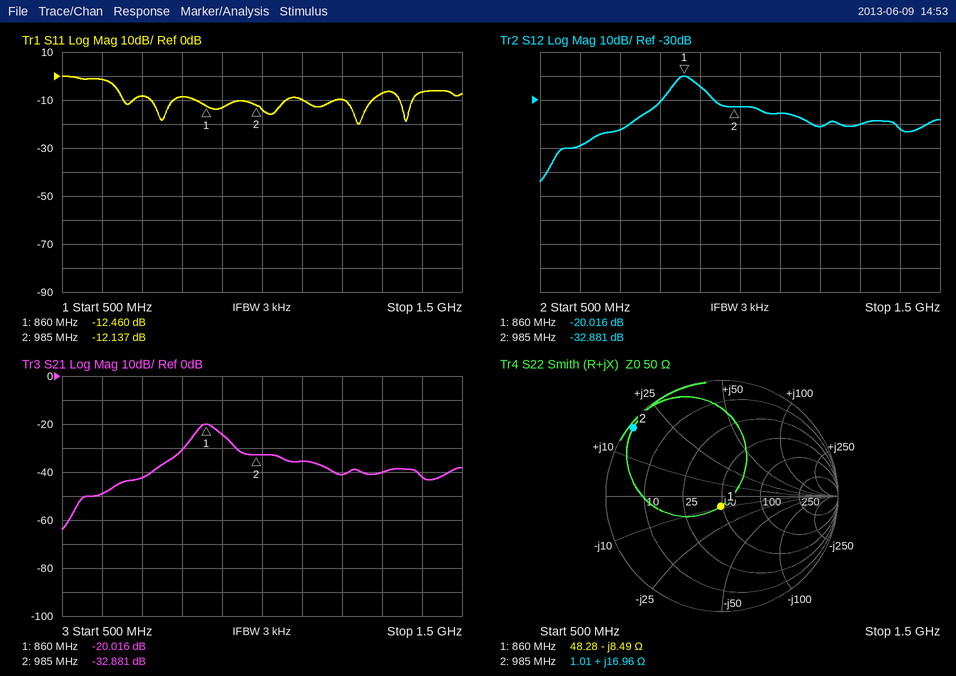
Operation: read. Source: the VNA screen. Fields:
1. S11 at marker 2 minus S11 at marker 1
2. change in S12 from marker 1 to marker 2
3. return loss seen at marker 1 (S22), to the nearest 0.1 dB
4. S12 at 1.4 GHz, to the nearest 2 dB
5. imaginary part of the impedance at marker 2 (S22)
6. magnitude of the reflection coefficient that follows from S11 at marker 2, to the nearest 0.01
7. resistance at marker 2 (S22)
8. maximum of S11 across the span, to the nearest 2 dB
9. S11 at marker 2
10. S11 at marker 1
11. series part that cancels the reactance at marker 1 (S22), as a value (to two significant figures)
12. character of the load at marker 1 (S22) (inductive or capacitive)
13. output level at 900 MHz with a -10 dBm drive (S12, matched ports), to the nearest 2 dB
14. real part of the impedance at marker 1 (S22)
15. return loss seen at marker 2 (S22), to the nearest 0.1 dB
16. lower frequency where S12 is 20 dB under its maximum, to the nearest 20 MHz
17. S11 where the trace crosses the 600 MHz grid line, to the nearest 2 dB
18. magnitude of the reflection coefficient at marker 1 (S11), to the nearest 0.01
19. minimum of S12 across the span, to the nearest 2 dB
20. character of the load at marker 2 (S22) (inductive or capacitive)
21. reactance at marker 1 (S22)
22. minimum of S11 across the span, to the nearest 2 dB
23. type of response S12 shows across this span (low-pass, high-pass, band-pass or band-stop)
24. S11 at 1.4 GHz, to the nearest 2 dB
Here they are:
0.323 dB
-12.865 dB
21.1 dB
-42 dB
+16.96 Ω
0.25
1.01 Ω
0 dB
-12.137 dB
-12.460 dB
1.6 nH
capacitive
-34 dBm
48.28 Ω
0.3 dB
720 MHz
-2 dB
0.24
-64 dB
inductive
-8.49 Ω
-20 dB
band-pass
-6 dB
